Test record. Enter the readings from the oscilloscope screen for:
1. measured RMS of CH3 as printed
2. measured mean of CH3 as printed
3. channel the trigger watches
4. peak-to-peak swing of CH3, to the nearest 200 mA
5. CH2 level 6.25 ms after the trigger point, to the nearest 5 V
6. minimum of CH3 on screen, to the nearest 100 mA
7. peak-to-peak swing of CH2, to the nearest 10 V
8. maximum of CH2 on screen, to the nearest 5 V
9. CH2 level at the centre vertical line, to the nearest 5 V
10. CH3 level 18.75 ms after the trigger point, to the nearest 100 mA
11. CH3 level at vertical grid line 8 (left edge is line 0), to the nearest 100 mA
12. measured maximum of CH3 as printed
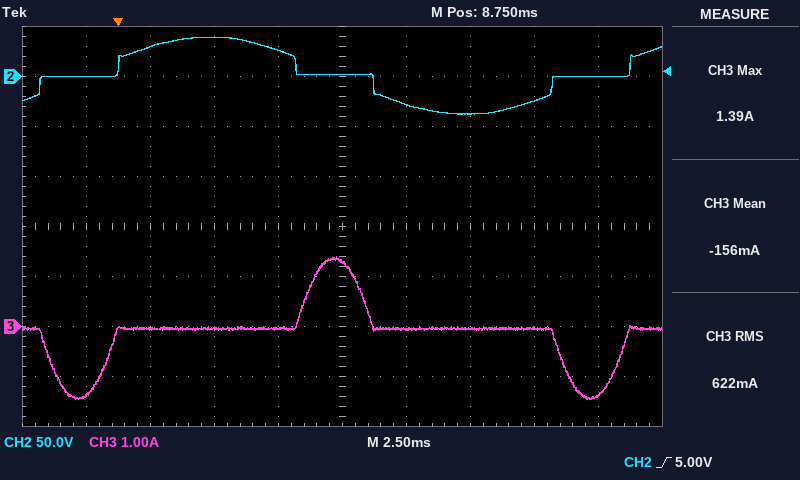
622 mA
-156 mA
CH2
2.8 A
25 V
-1.5 A
80 V
40 V
0 V
-1.4 A
0.0 A
1.39 A
